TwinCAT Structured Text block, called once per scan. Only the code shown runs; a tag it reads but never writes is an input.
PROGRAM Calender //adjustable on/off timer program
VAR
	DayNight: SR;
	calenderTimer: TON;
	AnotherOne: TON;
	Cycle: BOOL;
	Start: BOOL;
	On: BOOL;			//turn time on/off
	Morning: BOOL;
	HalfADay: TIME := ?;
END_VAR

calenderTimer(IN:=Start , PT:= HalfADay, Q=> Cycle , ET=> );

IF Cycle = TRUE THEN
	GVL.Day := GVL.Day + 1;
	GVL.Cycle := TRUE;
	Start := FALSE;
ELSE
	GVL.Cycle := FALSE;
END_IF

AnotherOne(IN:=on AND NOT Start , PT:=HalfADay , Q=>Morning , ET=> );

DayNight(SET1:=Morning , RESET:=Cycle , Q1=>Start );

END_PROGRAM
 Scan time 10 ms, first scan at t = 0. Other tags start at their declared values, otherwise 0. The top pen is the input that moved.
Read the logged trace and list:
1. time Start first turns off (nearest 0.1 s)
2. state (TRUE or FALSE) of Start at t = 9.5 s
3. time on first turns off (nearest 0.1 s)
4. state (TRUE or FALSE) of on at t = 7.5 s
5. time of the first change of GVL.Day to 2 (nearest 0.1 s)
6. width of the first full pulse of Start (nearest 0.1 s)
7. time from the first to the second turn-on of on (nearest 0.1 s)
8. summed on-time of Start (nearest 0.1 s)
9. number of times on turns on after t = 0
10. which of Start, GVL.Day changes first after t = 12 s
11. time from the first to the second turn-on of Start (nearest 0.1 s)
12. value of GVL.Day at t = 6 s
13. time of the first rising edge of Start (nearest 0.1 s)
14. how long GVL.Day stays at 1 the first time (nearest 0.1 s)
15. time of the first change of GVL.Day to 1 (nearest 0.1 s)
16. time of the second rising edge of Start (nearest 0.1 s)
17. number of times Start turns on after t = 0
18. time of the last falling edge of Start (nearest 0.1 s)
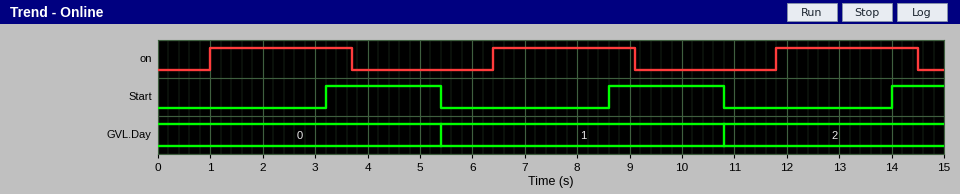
5.4 s
TRUE
3.7 s
TRUE
10.8 s
2.2 s
5.4 s
5.4 s
3
Start
5.4 s
1
3.2 s
5.4 s
5.4 s
8.6 s
3
10.8 s
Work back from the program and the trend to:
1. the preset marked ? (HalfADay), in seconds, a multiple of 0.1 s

2.2 s
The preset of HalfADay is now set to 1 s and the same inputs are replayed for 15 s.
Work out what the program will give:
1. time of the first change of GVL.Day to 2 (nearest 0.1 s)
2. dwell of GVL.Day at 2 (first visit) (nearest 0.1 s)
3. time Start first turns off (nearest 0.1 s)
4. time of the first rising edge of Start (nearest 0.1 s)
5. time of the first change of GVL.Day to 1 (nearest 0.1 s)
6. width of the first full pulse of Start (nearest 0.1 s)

8.4 s
5.4 s
3.0 s
2.0 s
3.0 s
1.0 s
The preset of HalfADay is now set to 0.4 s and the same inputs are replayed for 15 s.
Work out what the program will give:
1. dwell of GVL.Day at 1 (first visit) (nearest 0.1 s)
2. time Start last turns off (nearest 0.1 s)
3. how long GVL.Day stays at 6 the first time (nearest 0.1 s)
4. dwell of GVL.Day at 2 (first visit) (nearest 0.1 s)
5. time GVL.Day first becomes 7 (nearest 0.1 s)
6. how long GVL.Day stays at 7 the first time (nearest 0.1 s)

0.8 s
14.2 s
3.8 s
0.8 s
12.6 s
0.8 s
